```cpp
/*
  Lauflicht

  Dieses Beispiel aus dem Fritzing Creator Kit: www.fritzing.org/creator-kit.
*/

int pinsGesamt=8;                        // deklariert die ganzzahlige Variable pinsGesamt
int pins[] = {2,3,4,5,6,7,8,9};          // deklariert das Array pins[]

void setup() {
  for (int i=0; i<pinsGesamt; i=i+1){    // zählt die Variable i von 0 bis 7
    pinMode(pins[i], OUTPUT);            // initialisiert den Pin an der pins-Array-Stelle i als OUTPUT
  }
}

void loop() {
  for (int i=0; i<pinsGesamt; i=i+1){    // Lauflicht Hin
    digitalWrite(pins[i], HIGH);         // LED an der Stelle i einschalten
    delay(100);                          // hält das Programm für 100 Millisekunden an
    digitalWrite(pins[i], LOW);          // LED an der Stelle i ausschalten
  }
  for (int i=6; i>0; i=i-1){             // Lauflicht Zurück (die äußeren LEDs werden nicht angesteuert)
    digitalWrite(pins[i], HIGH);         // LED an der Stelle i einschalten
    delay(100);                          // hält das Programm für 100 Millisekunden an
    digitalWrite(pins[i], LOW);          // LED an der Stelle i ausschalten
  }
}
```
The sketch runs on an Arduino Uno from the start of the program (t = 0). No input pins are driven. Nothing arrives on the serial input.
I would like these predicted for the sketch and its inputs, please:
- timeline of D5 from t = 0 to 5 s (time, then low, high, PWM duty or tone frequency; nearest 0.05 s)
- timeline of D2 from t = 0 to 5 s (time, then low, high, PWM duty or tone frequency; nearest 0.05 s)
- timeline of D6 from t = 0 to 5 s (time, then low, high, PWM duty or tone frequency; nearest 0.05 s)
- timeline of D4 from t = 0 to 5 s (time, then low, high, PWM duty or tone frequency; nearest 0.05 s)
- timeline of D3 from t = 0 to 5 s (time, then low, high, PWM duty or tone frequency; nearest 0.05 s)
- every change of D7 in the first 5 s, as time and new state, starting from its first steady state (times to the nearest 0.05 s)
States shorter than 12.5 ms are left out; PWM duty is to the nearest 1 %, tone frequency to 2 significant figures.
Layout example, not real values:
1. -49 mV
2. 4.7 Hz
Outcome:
1. 0 s low; 0.3 s high; 0.4 s low; 1.1 s high; 1.2 s low; 1.7 s high; 1.8 s low; 2.5 s high; 2.6 s low; 3.1 s high; 3.2 s low; 3.9 s high; 4 s low; 4.5 s high; 4.6 s low
2. 0 s high; 0.1 s low; 1.4 s high; 1.5 s low; 2.8 s high; 2.9 s low; 4.2 s high; 4.3 s low
3. 0 s low; 0.4 s high; 0.5 s low; 1 s high; 1.1 s low; 1.8 s high; 1.9 s low; 2.4 s high; 2.5 s low; 3.2 s high; 3.3 s low; 3.8 s high; 3.9 s low; 4.6 s high; 4.7 s low
4. 0 s low; 0.2 s high; 0.3 s low; 1.2 s high; 1.3 s low; 1.6 s high; 1.7 s low; 2.6 s high; 2.7 s low; 3 s high; 3.1 s low; 4 s high; 4.1 s low; 4.4 s high; 4.5 s low
5. 0 s low; 0.1 s high; 0.2 s low; 1.3 s high; 1.4 s low; 1.5 s high; 1.6 s low; 2.7 s high; 2.8 s low; 2.9 s high; 3 s low; 4.1 s high; 4.2 s low; 4.3 s high; 4.4 s low
6. 0 s low; 0.5 s high; 0.6 s low; 0.9 s high; 1 s low; 1.9 s high; 2 s low; 2.3 s high; 2.4 s low; 3.3 s high; 3.4 s low; 3.7 s high; 3.8 s low; 4.7 s high; 4.8 s low
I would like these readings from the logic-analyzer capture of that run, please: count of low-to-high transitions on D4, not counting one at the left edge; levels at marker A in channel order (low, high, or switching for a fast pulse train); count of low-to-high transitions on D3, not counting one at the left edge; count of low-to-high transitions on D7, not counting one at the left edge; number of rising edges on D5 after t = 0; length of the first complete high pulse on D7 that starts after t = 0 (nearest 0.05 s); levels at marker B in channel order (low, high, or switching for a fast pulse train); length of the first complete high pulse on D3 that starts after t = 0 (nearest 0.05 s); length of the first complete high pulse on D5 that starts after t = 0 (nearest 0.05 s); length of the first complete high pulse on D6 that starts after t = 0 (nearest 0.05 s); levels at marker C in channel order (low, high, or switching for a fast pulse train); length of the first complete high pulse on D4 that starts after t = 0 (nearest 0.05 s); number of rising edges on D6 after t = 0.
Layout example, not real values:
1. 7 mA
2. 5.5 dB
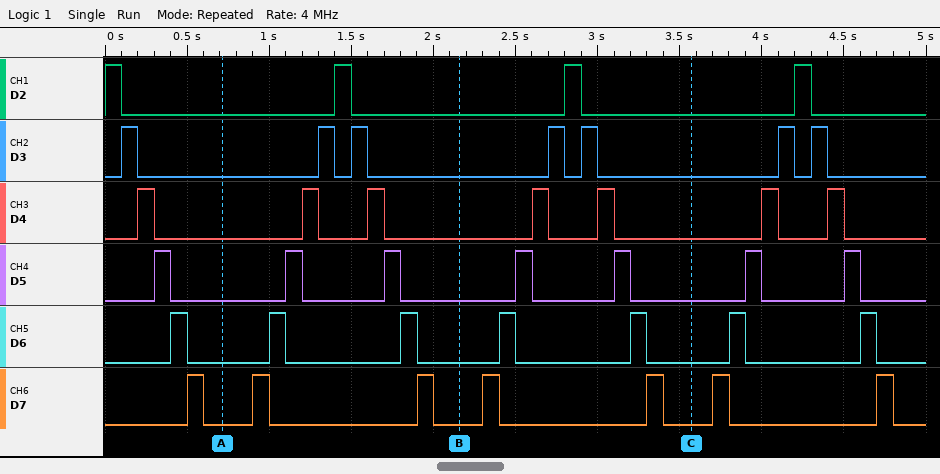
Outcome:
1. 7
2. D2 low, D3 low, D4 low, D5 low, D6 low, D7 low
3. 7
4. 7
5. 7
6. 0.10 s
7. D2 low, D3 low, D4 low, D5 low, D6 low, D7 low
8. 0.10 s
9. 0.10 s
10. 0.10 s
11. D2 low, D3 low, D4 low, D5 low, D6 low, D7 low
12. 0.10 s
13. 7
